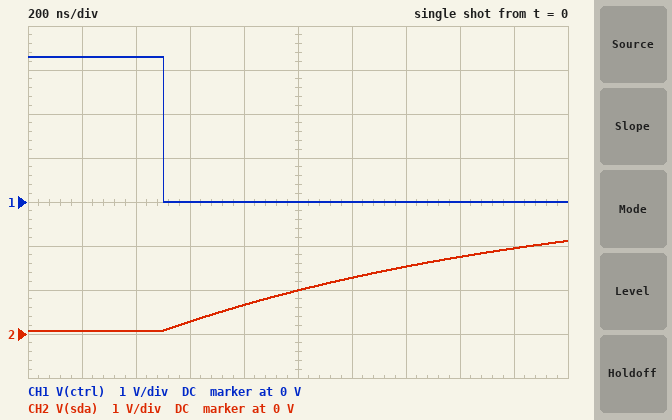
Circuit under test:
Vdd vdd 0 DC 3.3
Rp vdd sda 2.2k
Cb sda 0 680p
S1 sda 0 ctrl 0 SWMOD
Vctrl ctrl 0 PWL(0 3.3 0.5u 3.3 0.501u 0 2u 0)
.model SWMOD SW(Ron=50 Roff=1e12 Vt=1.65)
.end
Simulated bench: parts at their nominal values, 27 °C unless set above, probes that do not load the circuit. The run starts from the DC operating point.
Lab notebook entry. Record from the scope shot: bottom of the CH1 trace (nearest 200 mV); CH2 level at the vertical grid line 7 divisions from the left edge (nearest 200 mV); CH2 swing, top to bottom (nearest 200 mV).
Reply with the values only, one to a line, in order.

0 V
1.6 V
2.0 V
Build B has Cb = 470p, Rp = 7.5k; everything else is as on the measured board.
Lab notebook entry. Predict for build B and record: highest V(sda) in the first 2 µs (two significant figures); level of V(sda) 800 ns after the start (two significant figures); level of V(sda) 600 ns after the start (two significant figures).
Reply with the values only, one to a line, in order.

1.2 V
290 mV
110 mV
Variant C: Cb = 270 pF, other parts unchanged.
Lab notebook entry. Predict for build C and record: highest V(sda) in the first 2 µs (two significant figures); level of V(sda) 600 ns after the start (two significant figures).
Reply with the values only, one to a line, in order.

3.0 V
570 mV
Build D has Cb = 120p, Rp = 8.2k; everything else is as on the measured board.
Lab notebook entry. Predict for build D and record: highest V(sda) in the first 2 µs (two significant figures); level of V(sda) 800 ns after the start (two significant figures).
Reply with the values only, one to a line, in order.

2.6 V
880 mV
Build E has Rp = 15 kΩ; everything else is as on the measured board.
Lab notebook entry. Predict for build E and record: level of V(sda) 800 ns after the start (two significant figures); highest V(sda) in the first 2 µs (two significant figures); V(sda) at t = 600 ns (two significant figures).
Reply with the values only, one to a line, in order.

110 mV
460 mV
43 mV
